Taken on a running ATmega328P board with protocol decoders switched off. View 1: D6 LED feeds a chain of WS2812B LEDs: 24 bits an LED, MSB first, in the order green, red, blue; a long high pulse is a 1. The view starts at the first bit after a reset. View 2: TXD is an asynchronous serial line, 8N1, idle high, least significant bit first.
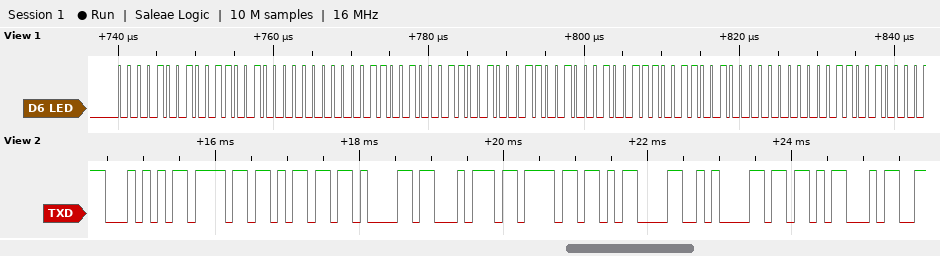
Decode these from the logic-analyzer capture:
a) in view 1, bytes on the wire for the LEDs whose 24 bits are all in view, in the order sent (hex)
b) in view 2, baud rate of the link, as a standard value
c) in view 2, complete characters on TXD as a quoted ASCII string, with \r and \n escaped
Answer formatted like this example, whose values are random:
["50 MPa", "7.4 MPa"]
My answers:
["09 32 00 32 32 32 27 32 00", "9600 baud", "\"Tomato\\r\\n[4\""]
